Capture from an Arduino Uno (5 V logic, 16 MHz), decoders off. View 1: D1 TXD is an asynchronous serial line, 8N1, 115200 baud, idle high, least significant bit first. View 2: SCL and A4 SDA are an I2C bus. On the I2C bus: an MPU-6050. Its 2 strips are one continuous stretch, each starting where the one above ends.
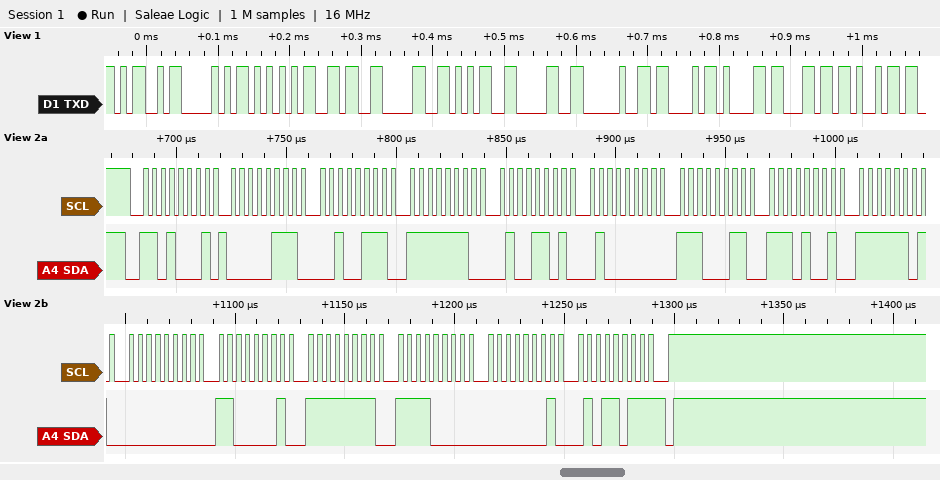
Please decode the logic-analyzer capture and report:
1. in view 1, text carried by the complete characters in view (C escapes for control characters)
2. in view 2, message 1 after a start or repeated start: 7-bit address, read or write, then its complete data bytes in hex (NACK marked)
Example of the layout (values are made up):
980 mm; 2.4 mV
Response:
"MPU6050 Cali"; 0x68 read: 07 27 FE 4D 40 E3 E9 FD 00 C1 FF F0 01 5B NACK
